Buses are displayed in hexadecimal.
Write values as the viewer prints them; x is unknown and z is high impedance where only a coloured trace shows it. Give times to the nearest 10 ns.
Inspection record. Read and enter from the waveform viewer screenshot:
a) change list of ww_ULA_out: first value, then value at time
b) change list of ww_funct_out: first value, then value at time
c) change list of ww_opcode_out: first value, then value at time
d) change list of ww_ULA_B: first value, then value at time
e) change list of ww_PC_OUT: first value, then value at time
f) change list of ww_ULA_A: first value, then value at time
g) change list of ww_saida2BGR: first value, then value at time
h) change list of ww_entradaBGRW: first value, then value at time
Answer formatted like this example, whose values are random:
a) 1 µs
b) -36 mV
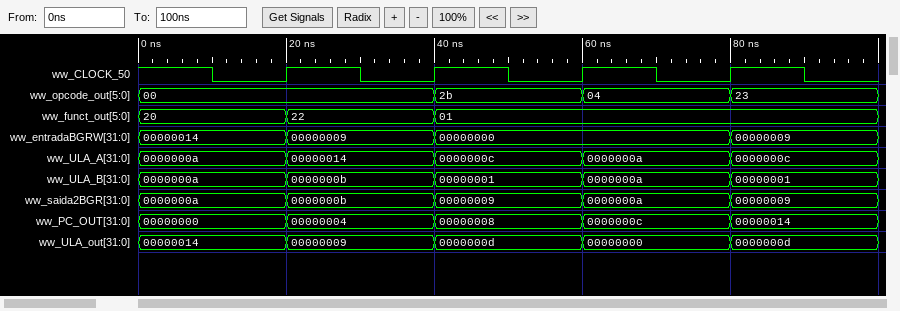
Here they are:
a) 00000014, 00000009 at 20 ns, 0000000d at 40 ns, 00000000 at 60 ns, 0000000d at 80 ns
b) 20, 22 at 20 ns, 01 at 40 ns
c) 00, 2b at 40 ns, 04 at 60 ns, 23 at 80 ns
d) 0000000a, 0000000b at 20 ns, 00000001 at 40 ns, 0000000a at 60 ns, 00000001 at 80 ns
e) 00000000, 00000004 at 20 ns, 00000008 at 40 ns, 0000000c at 60 ns, 00000014 at 80 ns
f) 0000000a, 00000014 at 20 ns, 0000000c at 40 ns, 0000000a at 60 ns, 0000000c at 80 ns
g) 0000000a, 0000000b at 20 ns, 00000009 at 40 ns, 0000000a at 60 ns, 00000009 at 80 ns
h) 00000014, 00000009 at 20 ns, 00000000 at 40 ns, 00000009 at 80 ns
